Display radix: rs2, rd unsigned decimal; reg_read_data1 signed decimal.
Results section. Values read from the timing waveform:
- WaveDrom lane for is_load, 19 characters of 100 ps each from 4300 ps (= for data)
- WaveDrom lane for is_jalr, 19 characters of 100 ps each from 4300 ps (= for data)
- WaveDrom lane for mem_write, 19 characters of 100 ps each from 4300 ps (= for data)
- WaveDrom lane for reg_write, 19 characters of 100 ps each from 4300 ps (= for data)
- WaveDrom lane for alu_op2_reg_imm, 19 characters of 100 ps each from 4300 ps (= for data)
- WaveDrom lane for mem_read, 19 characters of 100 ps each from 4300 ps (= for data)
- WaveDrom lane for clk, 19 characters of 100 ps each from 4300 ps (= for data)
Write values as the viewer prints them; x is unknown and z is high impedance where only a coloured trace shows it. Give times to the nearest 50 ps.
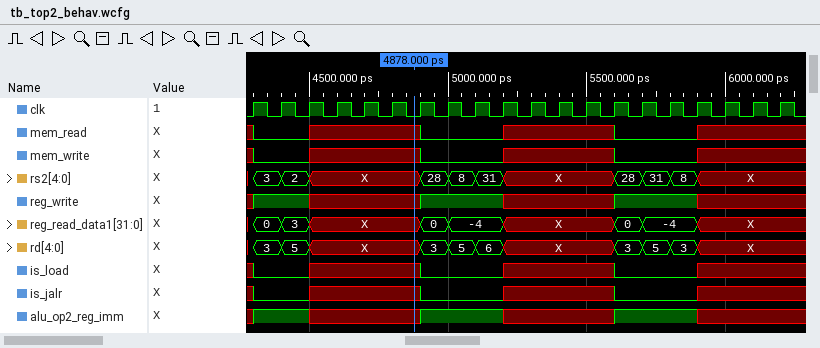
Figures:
{name: 'is_load', wave: '0.x...0..x...0..x..'}
{name: 'is_jalr', wave: '0.x...0..x...0..x..'}
{name: 'mem_write', wave: '0.x...0..x...0..x..'}
{name: 'reg_write', wave: '1.x...1..x...1..x..'}
{name: 'alu_op2_reg_imm', wave: '1.x...1..x...1..x..'}
{name: 'mem_read', wave: '0.x...0..x...0..x..'}
{name: 'clk', wave: 'p..................'}
